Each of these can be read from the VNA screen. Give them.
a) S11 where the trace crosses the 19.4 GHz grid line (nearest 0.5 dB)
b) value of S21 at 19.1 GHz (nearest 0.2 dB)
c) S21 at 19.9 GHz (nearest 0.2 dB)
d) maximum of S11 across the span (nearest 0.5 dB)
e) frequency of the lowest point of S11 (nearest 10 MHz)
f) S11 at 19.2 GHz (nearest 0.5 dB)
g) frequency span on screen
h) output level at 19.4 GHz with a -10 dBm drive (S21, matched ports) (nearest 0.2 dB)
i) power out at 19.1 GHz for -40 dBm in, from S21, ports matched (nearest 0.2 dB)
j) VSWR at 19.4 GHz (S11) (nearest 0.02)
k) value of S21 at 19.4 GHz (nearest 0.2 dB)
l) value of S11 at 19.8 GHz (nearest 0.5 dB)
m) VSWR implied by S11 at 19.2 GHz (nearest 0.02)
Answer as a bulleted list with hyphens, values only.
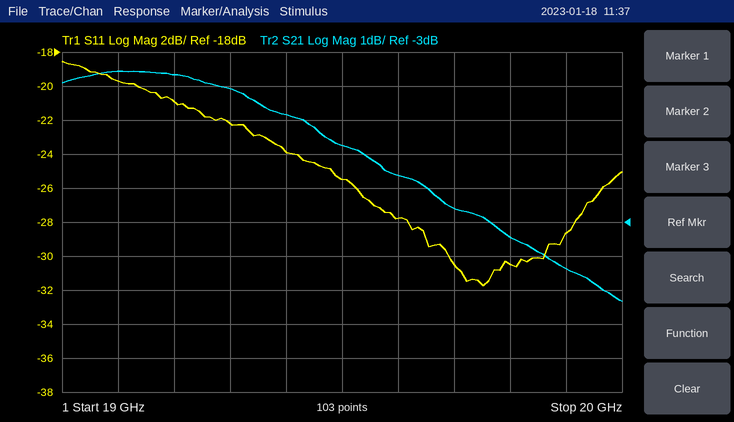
- -24.0 dB
- 1.4 dB
- -4.4 dB
- -18.5 dB
- 19.75 GHz
- -21.0 dB
- 1 GHz
- -9.8 dBm
- -38.6 dBm
- 1.14
- 0.2 dB
- -30.5 dB
- 1.20
